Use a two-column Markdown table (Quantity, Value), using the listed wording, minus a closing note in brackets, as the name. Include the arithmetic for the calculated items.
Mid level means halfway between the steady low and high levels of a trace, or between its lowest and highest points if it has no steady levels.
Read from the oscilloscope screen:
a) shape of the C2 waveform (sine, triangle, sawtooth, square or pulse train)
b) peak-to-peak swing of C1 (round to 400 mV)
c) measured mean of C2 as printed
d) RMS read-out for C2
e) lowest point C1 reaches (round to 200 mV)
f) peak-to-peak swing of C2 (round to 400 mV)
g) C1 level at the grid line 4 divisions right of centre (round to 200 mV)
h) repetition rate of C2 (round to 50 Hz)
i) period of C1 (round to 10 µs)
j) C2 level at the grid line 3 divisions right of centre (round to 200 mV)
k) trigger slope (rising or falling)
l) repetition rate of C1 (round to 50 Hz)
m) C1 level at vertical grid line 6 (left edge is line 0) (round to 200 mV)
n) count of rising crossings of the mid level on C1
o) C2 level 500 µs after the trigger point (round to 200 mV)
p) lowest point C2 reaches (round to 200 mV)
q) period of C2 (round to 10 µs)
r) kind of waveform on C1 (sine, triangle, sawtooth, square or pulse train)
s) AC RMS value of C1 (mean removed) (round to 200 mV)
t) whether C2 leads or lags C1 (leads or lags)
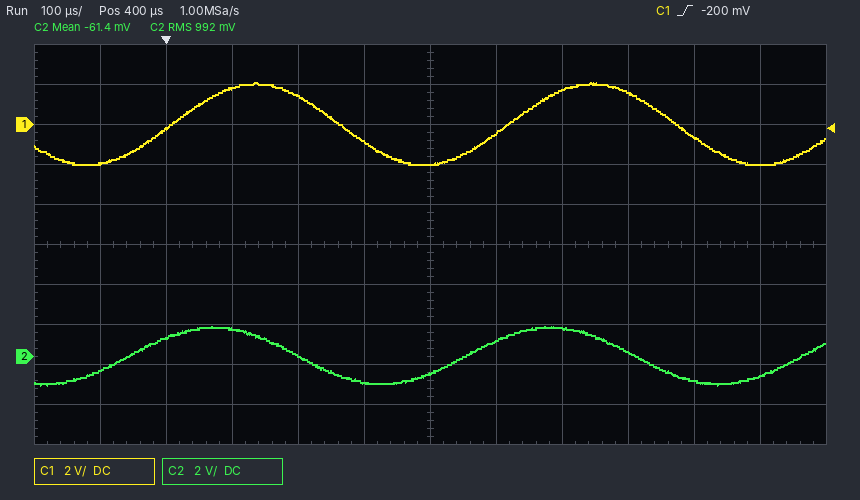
| Quantity | Value |
|---|---|
| shape of the C2 waveform | sine |
| peak-to-peak swing of C1 | 4.0 V |
| measured mean of C2 as printed | -61.4 mV |
| RMS read-out for C2 | 992 mV |
| lowest point C1 reaches | -2.0 V |
| peak-to-peak swing of C2 | 2.8 V |
| C1 level at the grid line 4 divisions right of centre | -600 mV |
| repetition rate of C2 | 1 / 510 µs ≈ 1.96 kHz, so 1.95 kHz to the nearest 50 Hz |
| period of C1 | 510 µs |
| C2 level at the grid line 3 divisions right of centre | 200 mV |
| trigger slope | rising |
| repetition rate of C1 | 1 / 510 µs ≈ 1.96 kHz, so 1.95 kHz to the nearest 50 Hz |
| C1 level at vertical grid line 6 (left edge is line 0) | -2.0 V |
| count of rising crossings of the mid level on C1 | 2 |
| C2 level 500 µs after the trigger point | 800 mV |
| lowest point C2 reaches | -1.4 V |
| period of C2 | 510 µs |
| kind of waveform on C1 | sine |
| AC RMS value of C1 (mean removed) | 4.0 V / (2√2) ≈ 1.4 V |
| whether C2 leads or lags C1 | leads |
